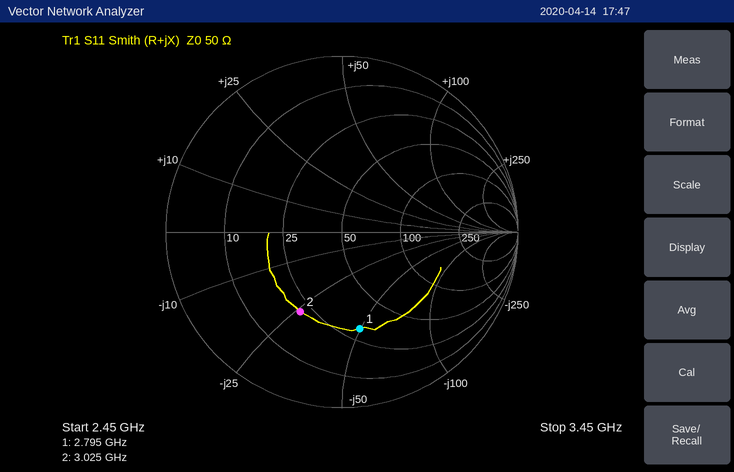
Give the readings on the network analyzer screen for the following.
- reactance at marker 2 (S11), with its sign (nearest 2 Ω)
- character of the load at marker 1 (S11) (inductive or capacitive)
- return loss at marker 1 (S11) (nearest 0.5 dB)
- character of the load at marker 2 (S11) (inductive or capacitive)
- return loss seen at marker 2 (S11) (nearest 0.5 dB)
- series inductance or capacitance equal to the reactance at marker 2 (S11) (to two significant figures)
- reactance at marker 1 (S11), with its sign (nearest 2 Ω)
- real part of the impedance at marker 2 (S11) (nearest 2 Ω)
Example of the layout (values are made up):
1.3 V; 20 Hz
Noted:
-26 Ω; capacitive; 5.0 dB; capacitive; 6.0 dB; 2.0 pF; -50 Ω; 22 Ω
